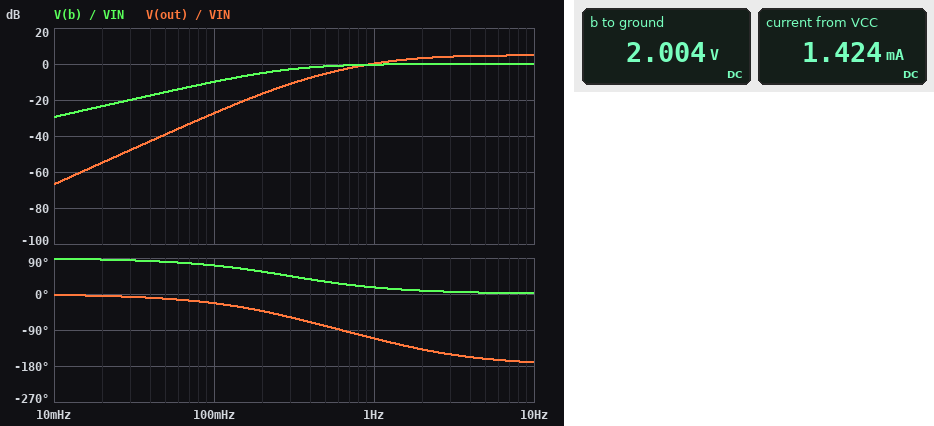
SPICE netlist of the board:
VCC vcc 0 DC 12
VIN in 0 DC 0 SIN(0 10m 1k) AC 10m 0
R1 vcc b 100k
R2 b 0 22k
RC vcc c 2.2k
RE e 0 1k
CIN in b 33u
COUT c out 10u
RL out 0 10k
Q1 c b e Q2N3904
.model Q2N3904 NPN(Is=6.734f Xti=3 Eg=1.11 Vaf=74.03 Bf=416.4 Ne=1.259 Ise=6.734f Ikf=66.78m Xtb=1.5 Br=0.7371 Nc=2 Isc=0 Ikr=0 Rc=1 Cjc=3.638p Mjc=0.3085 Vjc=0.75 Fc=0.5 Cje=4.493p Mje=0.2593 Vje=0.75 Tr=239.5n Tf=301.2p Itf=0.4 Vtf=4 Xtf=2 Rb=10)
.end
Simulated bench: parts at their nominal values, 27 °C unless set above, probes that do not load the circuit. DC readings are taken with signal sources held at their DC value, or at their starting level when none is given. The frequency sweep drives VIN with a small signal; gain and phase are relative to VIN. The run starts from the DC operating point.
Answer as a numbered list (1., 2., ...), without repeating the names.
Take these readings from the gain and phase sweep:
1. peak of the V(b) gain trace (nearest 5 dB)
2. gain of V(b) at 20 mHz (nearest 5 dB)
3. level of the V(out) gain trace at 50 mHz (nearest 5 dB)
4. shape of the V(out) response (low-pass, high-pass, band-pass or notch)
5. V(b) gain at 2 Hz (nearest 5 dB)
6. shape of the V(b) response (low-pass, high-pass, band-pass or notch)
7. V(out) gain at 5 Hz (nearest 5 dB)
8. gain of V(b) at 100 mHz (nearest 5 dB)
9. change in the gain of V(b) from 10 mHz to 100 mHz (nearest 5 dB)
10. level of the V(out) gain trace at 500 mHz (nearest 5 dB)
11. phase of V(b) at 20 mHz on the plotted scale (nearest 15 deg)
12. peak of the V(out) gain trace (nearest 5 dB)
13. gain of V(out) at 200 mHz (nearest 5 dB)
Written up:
1. 0 dB
2. -25 dB
3. -40 dB
4. high-pass
5. 0 dB
6. high-pass
7. 5 dB
8. -10 dB
9. 20 dB
10. -5 dB
11. 90 deg
12. 5 dB
13. -15 dB
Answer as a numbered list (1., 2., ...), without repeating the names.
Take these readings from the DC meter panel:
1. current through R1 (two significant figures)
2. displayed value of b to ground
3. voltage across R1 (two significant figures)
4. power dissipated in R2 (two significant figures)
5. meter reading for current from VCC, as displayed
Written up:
1. 100 µA
2. 2.004 V
3. 10 V
4. 180 µW
5. 1.424 mA
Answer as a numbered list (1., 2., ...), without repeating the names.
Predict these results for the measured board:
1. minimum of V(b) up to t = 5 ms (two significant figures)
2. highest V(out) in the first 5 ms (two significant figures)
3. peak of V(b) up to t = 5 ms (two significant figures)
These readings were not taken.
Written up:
1. 2.0 V
2. 18 mV
3. 2.0 V
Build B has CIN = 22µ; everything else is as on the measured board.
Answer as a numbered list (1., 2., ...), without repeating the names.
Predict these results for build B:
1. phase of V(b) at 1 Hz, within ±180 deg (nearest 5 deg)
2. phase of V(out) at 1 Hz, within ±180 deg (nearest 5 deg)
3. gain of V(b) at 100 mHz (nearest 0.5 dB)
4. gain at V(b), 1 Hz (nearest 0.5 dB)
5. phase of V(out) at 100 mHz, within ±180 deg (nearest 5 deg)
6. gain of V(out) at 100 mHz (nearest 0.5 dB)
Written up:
1. 25 deg
2. -105 deg
3. -13.0 dB
4. -1.0 dB
5. -15 deg
6. -30.5 dB
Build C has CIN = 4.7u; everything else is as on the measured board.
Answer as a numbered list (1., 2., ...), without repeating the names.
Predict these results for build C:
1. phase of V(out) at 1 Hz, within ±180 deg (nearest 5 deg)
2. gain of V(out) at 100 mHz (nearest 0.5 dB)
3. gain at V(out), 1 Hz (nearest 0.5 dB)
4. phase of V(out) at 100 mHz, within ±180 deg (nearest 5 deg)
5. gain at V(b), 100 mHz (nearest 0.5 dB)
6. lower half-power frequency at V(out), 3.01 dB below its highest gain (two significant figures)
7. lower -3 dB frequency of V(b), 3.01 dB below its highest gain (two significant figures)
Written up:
1. -65 deg
2. -44.0 dB
3. -6.5 dB
4. -5 deg
5. -26.5 dB
6. 2.7 Hz
7. 2.1 Hz
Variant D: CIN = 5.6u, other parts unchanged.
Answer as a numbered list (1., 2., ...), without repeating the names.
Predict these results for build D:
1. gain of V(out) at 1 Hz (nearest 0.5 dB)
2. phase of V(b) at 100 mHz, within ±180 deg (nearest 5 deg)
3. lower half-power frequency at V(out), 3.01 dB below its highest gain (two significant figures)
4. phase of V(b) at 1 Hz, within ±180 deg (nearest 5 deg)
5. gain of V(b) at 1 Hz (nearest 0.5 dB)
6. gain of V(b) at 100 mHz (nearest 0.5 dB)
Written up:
1. -5.5 dB
2. 85 deg
3. 2.4 Hz
4. 60 deg
5. -6.0 dB
6. -25.0 dB
